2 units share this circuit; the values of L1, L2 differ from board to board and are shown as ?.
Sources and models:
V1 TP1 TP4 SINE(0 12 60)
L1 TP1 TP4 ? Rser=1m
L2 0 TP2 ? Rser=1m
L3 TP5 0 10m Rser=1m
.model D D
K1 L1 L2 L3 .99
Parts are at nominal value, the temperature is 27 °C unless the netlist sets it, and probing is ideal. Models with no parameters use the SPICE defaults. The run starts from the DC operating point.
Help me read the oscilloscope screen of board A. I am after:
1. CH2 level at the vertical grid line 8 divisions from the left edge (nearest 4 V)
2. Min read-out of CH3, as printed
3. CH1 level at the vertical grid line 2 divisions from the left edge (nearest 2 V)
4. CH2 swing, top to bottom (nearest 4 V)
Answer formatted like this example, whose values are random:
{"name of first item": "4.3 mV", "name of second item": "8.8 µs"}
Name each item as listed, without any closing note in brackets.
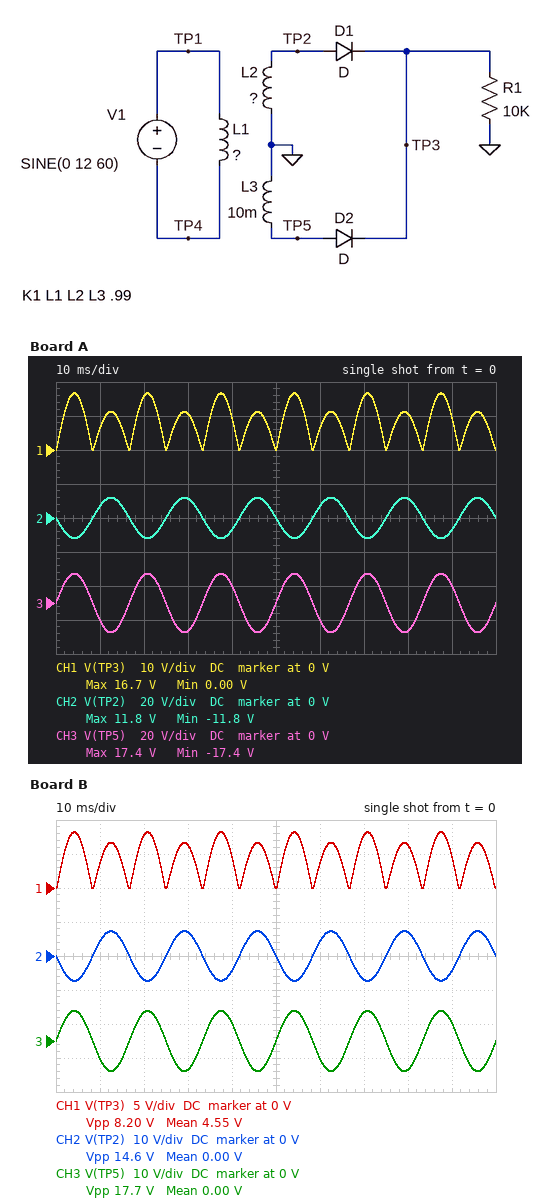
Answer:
{"CH2 level at the vertical grid line 8 divisions from the left edge": "12 V", "Min read-out of CH3, as printed": "-17.4 V", "CH1 level at the vertical grid line 2 divisions from the left edge": "16 V", "CH2 swing, top to bottom": "24 V"}
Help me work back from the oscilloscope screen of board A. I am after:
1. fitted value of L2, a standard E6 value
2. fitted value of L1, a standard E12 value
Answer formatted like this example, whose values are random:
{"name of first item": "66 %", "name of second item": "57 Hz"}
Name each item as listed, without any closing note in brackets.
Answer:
{"fitted value of L2, a standard E6 value": "4.7 mH", "fitted value of L1, a standard E12 value": "4.7 mH"}
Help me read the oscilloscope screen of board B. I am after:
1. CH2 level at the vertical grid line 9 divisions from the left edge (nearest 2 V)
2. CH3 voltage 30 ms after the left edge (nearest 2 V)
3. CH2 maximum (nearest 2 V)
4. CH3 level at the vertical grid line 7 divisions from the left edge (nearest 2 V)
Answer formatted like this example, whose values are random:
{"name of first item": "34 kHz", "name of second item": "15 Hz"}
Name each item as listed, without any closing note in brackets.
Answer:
{"CH2 level at the vertical grid line 9 divisions from the left edge": "-4 V", "CH3 voltage 30 ms after the left edge": "-8 V", "CH2 maximum": "8 V", "CH3 level at the vertical grid line 7 divisions from the left edge": "8 V"}
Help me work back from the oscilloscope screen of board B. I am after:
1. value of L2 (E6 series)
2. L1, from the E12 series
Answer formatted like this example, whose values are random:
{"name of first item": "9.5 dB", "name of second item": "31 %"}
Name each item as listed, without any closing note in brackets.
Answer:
{"value of L2": "6.8 mH", "L1, from the E12 series": "18 mH"}
